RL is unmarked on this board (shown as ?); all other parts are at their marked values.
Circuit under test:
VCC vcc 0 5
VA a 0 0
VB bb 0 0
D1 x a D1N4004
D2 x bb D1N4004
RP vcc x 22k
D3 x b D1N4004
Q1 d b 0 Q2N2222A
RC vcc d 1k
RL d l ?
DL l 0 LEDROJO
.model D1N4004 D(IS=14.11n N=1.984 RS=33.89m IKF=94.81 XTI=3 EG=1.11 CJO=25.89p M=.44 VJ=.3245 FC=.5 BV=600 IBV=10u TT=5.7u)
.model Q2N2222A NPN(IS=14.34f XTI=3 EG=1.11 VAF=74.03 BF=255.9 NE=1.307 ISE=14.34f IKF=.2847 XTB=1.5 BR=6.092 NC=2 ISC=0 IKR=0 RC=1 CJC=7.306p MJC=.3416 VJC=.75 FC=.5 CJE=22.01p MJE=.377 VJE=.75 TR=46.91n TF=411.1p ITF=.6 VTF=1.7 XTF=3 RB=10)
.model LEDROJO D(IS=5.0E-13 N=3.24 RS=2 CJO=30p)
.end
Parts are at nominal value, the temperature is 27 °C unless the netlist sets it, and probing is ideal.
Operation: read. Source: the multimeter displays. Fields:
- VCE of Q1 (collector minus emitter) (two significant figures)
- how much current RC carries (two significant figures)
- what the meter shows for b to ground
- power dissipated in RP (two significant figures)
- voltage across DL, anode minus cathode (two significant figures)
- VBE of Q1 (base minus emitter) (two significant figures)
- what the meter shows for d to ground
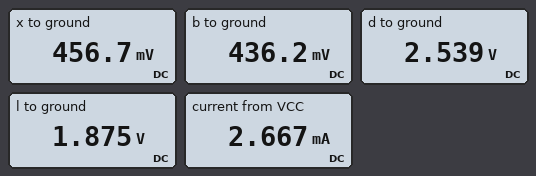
2.5 V
2.5 mA
436.2 mV
940 µW
1.9 V
440 mV
2.539 V
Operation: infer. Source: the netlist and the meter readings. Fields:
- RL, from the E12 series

270 Ω
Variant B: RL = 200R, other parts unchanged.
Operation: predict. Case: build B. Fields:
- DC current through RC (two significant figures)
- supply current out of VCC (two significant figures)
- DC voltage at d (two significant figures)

2.6 mA
2.8 mA
2.4 V
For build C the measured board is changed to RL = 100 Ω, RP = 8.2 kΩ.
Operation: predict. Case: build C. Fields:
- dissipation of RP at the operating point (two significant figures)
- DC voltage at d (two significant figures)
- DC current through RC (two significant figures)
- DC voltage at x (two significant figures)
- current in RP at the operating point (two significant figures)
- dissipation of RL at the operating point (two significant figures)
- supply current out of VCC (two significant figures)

2.5 mW
2.2 V
2.8 mA
510 mV
550 µA
800 µW
3.4 mA
